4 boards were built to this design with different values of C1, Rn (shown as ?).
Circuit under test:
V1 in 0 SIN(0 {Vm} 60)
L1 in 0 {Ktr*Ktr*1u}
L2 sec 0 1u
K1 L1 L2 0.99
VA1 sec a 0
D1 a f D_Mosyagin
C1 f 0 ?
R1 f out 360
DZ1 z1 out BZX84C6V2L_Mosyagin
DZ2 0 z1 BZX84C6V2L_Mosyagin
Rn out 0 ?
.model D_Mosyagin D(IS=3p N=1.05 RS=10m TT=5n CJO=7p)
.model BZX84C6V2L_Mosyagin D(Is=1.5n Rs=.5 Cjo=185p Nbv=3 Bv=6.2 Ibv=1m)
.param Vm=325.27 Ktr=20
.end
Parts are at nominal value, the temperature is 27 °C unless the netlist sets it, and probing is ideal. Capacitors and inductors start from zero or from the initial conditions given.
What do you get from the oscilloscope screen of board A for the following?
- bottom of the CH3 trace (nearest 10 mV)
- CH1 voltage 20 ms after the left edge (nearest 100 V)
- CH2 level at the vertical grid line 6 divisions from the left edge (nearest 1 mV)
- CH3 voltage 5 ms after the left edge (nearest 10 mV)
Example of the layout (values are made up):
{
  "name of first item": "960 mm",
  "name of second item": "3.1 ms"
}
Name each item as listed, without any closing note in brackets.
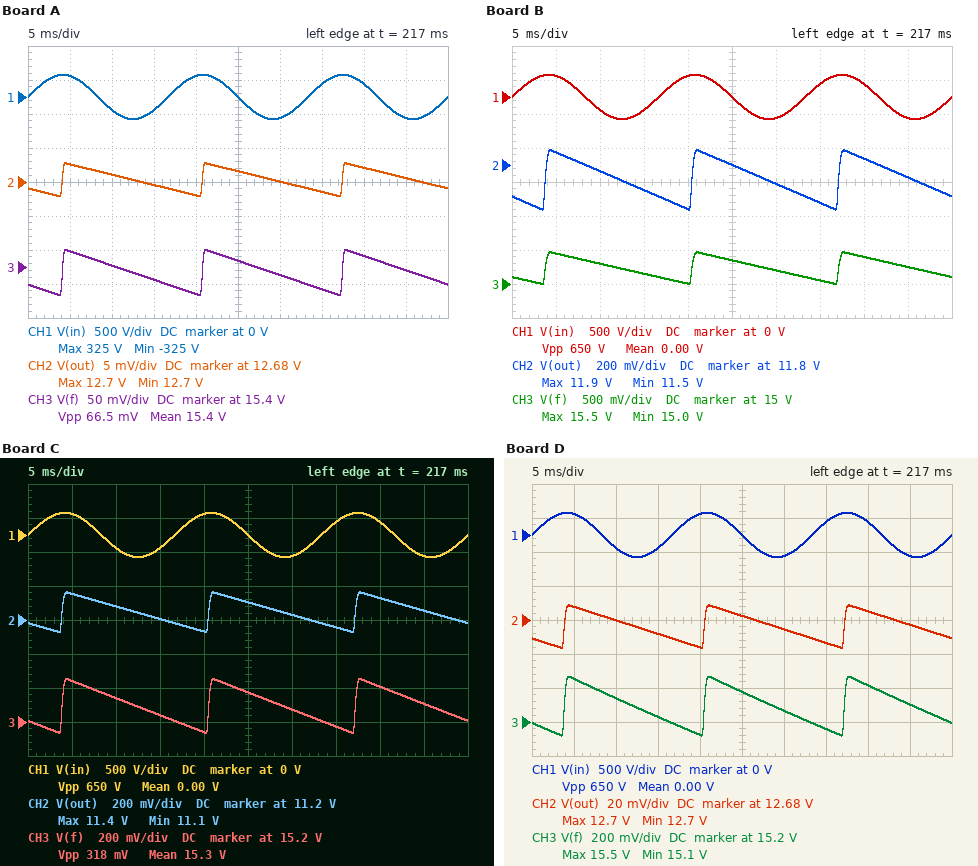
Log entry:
{
  "bottom of the CH3 trace": "15.36 V",
  "CH1 voltage 20 ms after the left edge": "300 V",
  "CH2 level at the vertical grid line 6 divisions from the left edge": "12.675 V",
  "CH3 voltage 5 ms after the left edge": "15.42 V"
}
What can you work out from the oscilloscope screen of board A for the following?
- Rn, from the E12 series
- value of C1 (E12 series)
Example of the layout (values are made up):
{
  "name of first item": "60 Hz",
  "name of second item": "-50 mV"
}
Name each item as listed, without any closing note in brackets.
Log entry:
{
  "Rn, from the E12 series": "6.8 kΩ",
  "value of C1": "1.8 mF"
}
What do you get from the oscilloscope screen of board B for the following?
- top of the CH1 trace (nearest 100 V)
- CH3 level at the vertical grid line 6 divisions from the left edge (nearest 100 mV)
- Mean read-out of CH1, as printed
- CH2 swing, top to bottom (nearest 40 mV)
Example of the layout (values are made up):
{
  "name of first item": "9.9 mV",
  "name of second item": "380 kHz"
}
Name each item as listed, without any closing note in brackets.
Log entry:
{
  "top of the CH1 trace": "300 V",
  "CH3 level at the vertical grid line 6 divisions from the left edge": "15.2 V",
  "Mean read-out of CH1, as printed": "0.00 V",
  "CH2 swing, top to bottom": "360 mV"
}
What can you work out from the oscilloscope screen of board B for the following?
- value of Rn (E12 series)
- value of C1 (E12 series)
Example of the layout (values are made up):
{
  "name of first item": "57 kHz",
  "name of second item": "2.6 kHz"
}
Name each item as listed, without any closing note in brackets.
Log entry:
{
  "value of Rn": "1.2 kΩ",
  "value of C1": "330 µF"
}
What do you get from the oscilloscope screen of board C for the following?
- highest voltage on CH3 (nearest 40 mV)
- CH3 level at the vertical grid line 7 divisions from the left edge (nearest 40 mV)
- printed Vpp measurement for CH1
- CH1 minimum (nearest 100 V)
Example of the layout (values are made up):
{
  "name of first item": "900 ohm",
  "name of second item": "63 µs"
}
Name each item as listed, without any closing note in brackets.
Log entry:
{
  "highest voltage on CH3": "15.44 V",
  "CH3 level at the vertical grid line 7 divisions from the left edge": "15.16 V",
  "printed Vpp measurement for CH1": "650 V",
  "CH1 minimum": "-300 V"
}
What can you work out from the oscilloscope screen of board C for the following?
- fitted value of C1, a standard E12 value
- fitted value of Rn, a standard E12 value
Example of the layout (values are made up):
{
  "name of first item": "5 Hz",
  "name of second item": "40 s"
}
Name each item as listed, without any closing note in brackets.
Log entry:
{
  "fitted value of C1, a standard E12 value": "560 µF",
  "fitted value of Rn, a standard E12 value": "1 kΩ"
}
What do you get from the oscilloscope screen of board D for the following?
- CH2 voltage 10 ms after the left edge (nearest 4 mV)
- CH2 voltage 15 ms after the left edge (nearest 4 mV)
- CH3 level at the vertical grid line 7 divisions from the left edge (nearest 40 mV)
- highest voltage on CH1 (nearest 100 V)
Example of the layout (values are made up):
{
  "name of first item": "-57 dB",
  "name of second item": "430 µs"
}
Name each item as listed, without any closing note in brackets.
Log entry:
{
  "CH2 voltage 10 ms after the left edge": "12.680 V",
  "CH2 voltage 15 ms after the left edge": "12.672 V",
  "CH3 level at the vertical grid line 7 divisions from the left edge": "15.16 V",
  "highest voltage on CH1": "300 V"
}
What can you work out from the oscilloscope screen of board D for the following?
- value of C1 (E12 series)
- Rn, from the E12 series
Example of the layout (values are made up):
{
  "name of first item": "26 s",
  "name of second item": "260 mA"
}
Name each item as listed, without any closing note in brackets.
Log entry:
{
  "value of C1": "330 µF",
  "Rn, from the E12 series": "8.2 kΩ"
}
